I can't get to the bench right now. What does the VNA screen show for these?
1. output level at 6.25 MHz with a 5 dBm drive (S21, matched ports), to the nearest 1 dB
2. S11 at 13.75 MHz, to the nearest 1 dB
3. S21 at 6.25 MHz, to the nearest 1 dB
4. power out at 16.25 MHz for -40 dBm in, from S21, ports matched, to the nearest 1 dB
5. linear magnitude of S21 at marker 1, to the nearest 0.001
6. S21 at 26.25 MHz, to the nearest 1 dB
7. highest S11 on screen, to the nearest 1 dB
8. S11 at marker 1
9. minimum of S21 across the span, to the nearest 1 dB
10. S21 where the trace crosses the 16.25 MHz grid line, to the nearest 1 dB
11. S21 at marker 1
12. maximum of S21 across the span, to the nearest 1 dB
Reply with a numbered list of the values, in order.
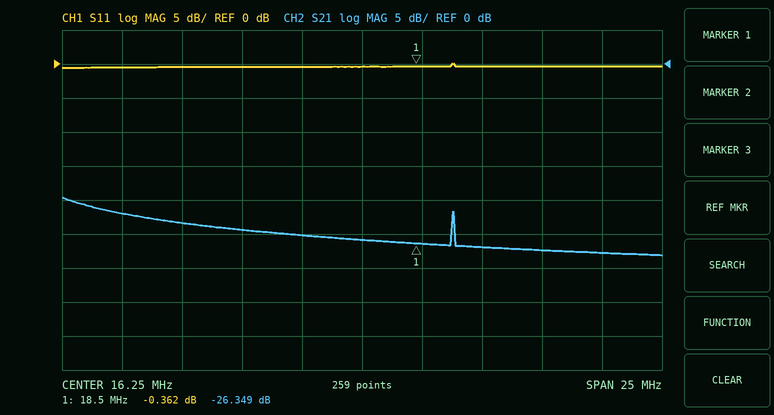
1. -17 dBm
2. 0 dB
3. -22 dB
4. -66 dBm
5. 0.048
6. -28 dB
7. 0 dB
8. -0.362 dB
9. -28 dB
10. -26 dB
11. -26.349 dB
12. -20 dB
